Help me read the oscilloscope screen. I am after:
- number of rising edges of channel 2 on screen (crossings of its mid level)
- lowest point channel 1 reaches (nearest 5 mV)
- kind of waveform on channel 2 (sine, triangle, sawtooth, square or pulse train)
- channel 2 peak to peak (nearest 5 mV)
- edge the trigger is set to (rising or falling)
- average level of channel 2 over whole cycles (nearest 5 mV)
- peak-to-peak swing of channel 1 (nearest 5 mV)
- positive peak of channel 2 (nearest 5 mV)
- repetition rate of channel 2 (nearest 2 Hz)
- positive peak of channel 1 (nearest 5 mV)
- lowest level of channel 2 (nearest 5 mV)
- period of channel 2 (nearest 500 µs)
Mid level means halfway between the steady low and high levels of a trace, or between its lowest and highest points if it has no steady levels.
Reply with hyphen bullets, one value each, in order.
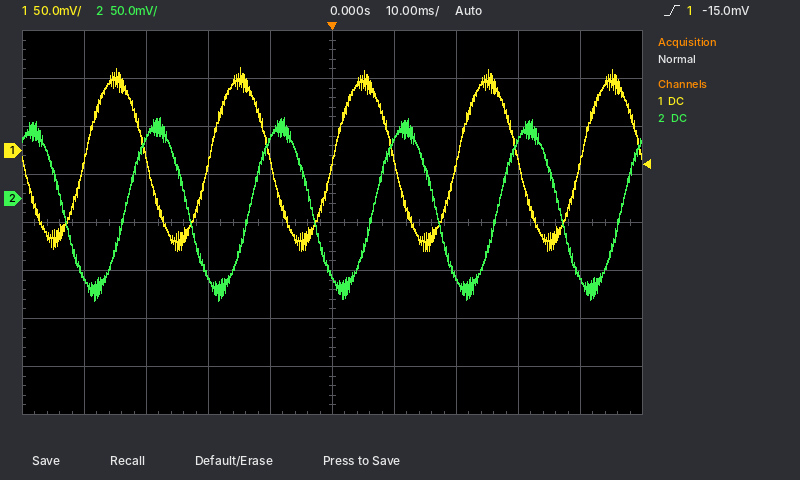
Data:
- 5
- -105 mV
- sine
- 190 mV
- rising
- -10 mV
- 190 mV
- 85 mV
- 50 Hz
- 85 mV
- -105 mV
- 20.0 ms
